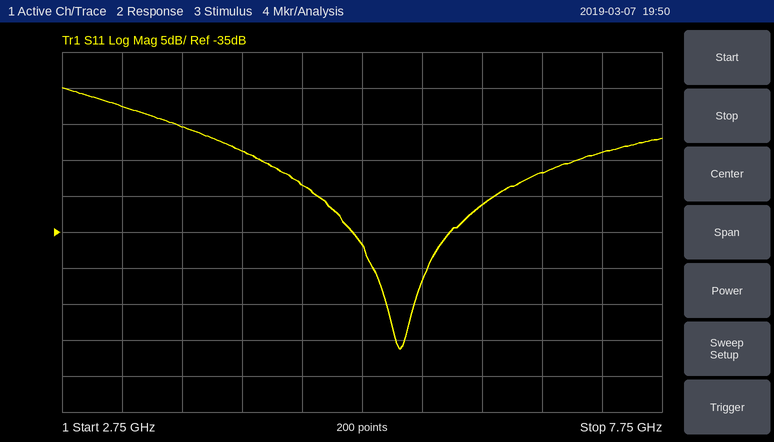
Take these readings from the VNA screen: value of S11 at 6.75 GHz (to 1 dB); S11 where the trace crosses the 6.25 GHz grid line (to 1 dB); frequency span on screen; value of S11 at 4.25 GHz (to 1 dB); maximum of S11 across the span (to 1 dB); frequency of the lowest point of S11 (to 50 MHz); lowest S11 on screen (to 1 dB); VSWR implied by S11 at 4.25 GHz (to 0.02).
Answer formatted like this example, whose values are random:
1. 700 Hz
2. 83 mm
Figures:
1. -27 dB
2. -31 dB
3. 5 GHz
4. -24 dB
5. -15 dB
6. 5.55 GHz
7. -51 dB
8. 1.14
